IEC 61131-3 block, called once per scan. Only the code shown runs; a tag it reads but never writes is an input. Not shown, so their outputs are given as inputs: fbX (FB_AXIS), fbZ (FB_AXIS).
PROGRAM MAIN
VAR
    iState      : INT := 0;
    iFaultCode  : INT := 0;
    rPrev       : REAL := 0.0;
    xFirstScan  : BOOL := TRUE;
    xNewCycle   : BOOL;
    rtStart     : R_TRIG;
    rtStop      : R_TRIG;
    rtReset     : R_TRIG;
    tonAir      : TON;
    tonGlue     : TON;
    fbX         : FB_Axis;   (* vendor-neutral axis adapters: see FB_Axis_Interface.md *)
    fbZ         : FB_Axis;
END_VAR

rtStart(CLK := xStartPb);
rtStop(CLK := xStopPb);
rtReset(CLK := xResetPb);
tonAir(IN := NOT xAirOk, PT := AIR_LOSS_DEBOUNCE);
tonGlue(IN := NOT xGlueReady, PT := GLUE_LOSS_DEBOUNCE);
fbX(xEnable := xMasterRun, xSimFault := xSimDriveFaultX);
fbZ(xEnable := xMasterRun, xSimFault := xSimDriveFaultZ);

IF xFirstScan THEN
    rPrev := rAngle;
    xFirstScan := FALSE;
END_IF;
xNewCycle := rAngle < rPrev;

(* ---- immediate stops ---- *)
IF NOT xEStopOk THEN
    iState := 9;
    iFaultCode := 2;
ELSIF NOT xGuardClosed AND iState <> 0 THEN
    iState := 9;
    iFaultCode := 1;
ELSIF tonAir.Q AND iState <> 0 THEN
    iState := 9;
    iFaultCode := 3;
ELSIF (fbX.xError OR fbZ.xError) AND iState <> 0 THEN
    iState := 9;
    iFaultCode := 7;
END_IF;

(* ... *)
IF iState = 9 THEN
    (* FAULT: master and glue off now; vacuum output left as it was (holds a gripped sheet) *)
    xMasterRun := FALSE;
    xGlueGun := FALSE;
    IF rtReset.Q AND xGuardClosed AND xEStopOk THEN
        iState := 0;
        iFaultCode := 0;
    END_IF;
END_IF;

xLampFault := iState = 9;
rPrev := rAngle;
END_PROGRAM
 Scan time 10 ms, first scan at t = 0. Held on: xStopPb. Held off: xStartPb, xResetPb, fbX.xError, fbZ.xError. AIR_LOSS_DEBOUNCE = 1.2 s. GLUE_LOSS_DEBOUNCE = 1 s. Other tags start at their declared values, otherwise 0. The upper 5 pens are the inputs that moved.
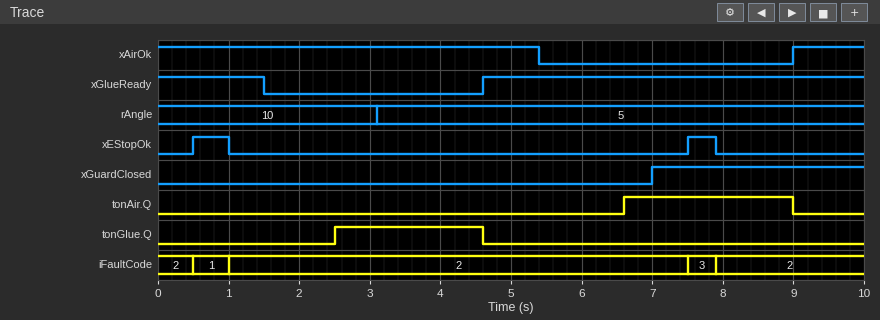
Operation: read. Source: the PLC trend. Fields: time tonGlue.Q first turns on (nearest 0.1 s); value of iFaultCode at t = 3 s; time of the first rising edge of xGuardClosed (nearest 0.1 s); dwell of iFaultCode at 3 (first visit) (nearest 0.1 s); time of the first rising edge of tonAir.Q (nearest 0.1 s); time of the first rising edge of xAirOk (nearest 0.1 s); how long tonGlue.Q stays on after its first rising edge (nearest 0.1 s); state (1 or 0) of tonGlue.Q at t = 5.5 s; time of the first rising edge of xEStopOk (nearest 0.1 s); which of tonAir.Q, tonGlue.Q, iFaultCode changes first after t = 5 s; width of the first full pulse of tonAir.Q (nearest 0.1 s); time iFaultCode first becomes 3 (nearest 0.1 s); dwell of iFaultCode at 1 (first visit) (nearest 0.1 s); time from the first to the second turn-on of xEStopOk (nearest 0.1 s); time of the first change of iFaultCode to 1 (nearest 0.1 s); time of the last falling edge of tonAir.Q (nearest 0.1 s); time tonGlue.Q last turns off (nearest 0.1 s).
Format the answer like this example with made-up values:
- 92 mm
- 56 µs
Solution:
- 2.5 s
- 2
- 7.0 s
- 0.4 s
- 6.6 s
- 9.0 s
- 2.1 s
- 0
- 0.5 s
- tonAir.Q
- 2.4 s
- 7.5 s
- 0.5 s
- 7.0 s
- 0.5 s
- 9.0 s
- 4.6 s
